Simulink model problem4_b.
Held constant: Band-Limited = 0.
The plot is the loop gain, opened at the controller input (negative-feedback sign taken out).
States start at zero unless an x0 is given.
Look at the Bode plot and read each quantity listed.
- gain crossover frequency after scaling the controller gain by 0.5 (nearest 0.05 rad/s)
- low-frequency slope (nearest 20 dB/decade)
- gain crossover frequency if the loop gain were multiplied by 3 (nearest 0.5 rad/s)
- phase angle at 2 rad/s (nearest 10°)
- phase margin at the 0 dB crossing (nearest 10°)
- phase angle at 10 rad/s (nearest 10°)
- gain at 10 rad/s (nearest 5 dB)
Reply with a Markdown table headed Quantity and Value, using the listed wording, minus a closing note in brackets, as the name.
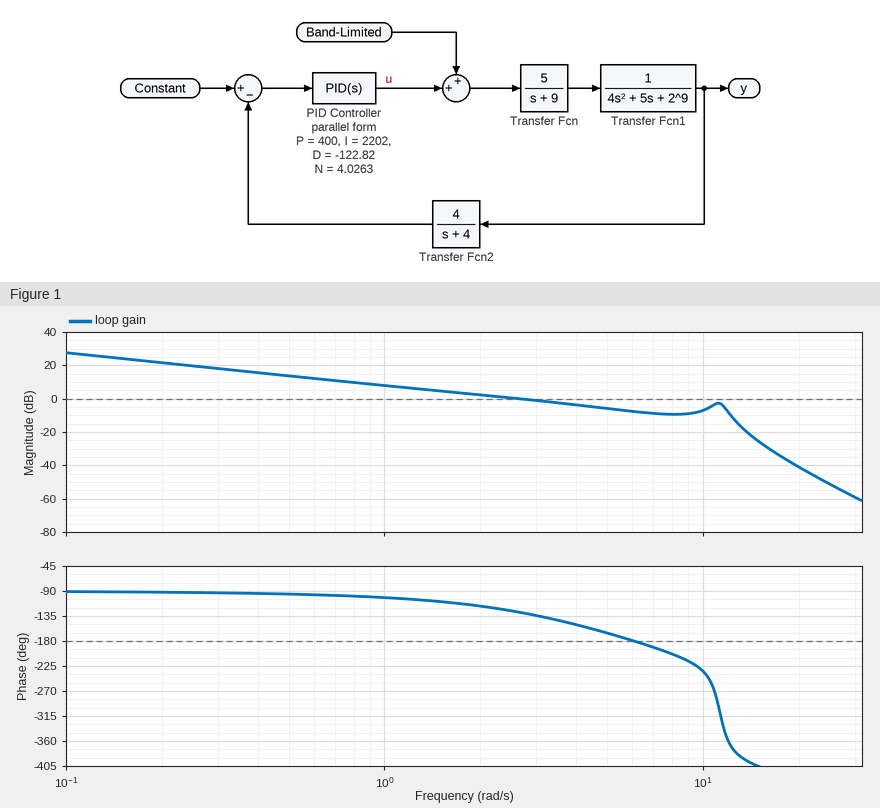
| Quantity | Value |
|---|---|
| gain crossover frequency after scaling the controller gain by 0.5 | 1.25 rad/s |
| low-frequency slope | -20 dB/decade |
| gain crossover frequency if the loop gain were multiplied by 3 | 12.0 rad/s |
| phase angle at 2 rad/s | -120° |
| phase margin at the 0 dB crossing | 50° |
| phase angle at 10 rad/s | -230° |
| gain at 10 rad/s | -5 dB |
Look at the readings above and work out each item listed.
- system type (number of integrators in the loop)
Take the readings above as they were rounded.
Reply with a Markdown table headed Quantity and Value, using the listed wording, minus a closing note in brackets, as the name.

| Quantity | Value |
|---|---|
| system type | 1 |
